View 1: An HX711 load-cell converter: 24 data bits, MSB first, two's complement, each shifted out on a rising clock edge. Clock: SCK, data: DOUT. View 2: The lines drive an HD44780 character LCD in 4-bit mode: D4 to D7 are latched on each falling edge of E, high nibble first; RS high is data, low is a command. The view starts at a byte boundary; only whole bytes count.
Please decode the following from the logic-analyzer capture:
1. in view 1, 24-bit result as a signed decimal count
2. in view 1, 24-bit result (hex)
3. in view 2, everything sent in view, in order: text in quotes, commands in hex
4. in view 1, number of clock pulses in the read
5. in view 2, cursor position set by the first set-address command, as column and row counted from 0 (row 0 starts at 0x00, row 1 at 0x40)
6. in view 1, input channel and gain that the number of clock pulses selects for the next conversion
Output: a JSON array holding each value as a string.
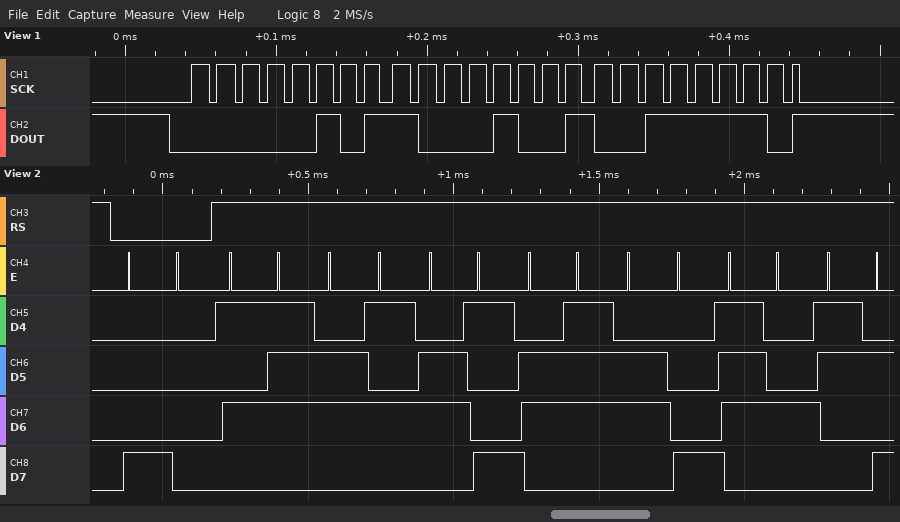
["362814", "0x05893E", "0x80 \"Weight:\"", "25", "column 0, row 0", "channel A, gain 128"]
